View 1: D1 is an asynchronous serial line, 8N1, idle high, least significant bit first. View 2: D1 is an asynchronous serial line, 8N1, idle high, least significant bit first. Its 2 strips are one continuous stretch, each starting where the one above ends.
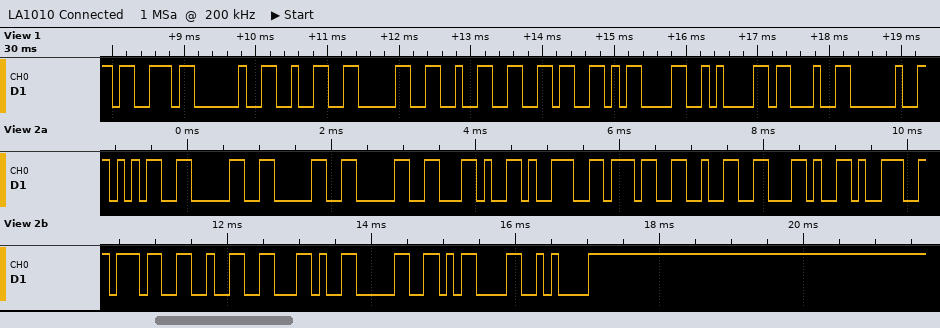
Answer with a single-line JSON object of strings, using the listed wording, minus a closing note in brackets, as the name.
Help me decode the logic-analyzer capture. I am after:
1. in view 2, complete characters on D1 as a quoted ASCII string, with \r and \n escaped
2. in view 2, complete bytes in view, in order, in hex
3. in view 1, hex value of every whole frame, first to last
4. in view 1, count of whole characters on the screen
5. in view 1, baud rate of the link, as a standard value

{"in view 2, complete characters on D1 as a quoted ASCII string, with \\r and \\n escaped": "\"5000,972,972,0\\r\\n\"", "in view 2, complete bytes in view, in order, in hex": "0x35 0x30 0x30 0x30 0x2C 0x39 0x37 0x32 0x2C 0x39 0x37 0x32 0x2C 0x30 0x0D 0x0A", "in view 1, hex value of every whole frame, first to last": "73 20 32 30 32 36 0D 0A 23 20", "in view 1, count of whole characters on the screen": "10", "in view 1, baud rate of the link, as a standard value": "9600 baud"}
